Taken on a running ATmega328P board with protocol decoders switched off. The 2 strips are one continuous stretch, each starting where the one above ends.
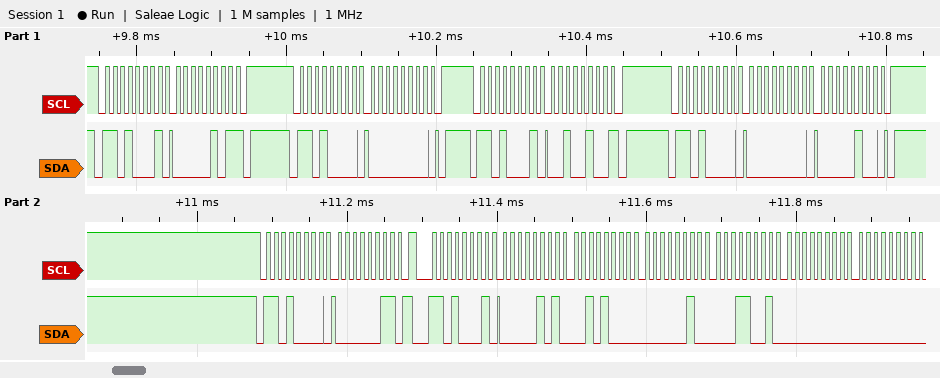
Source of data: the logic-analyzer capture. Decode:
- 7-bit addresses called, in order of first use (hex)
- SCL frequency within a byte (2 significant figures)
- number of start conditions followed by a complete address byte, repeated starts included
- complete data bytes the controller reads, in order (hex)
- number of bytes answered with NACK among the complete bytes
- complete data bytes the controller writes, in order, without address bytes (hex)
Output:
0x68
100 kHz
6
05 24 05 28 02 19 00 00
2
00 00 04 03
